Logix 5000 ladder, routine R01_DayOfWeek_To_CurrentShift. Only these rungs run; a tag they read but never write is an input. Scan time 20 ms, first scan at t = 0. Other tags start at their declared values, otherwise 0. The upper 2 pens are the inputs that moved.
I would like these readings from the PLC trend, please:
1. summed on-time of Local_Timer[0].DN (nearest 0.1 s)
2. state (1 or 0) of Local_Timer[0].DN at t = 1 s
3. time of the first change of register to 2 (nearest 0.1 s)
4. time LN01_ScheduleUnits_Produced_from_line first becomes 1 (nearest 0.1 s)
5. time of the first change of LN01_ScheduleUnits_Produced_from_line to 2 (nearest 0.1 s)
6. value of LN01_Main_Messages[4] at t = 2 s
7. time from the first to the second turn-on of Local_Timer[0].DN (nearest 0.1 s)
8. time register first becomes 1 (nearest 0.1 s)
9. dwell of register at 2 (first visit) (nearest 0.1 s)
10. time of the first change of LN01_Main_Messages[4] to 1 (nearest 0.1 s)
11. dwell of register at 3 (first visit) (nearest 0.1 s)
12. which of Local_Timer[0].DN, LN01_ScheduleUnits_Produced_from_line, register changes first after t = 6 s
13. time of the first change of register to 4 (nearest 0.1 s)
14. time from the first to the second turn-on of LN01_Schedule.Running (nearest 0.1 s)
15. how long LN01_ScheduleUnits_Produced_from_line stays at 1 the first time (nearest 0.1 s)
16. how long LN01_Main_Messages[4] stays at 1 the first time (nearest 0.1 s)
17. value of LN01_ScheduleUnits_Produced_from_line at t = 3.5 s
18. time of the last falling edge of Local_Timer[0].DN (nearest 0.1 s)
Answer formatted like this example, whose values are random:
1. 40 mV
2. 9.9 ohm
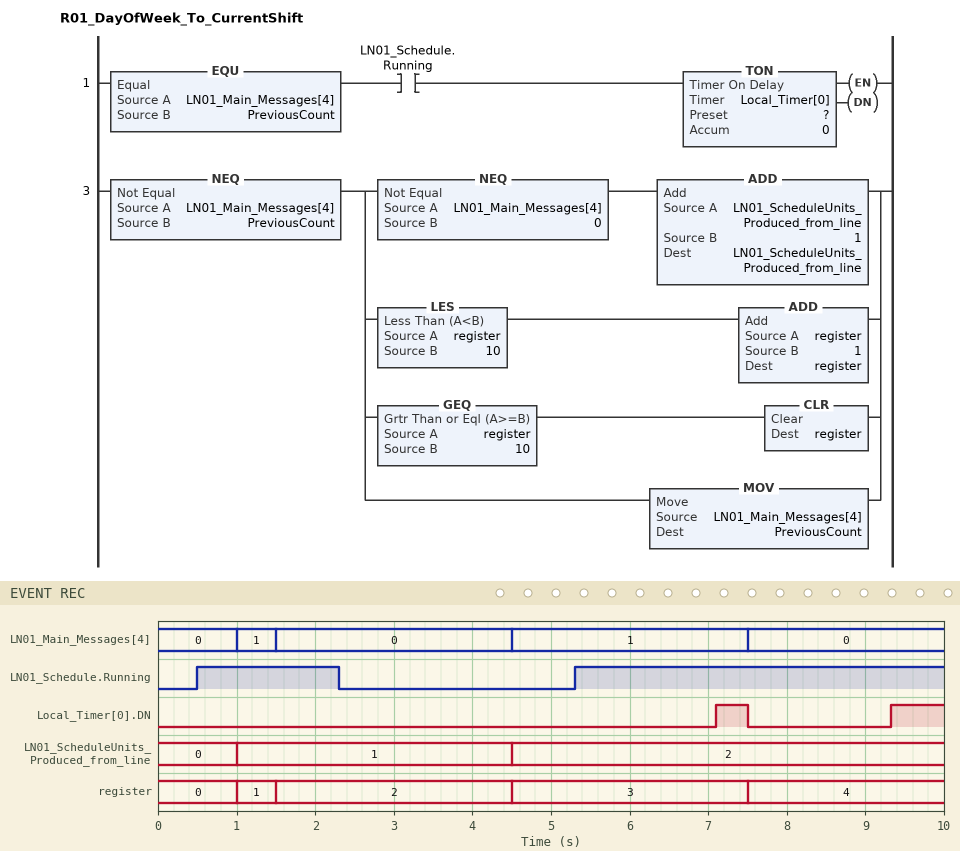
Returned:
1. 1.1 s
2. 0
3. 1.5 s
4. 1.0 s
5. 4.5 s
6. 0
7. 2.2 s
8. 1.0 s
9. 3.0 s
10. 1.0 s
11. 3.0 s
12. Local_Timer[0].DN
13. 7.5 s
14. 4.8 s
15. 3.5 s
16. 0.5 s
17. 1
18. 7.5 s
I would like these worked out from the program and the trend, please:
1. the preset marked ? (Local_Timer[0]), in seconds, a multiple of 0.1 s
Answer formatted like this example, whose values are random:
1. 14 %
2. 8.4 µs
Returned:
1. 1.8 s
